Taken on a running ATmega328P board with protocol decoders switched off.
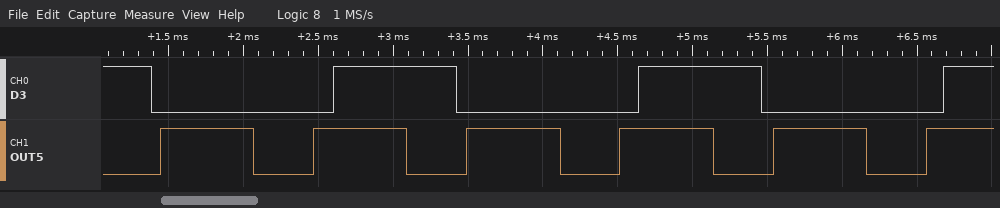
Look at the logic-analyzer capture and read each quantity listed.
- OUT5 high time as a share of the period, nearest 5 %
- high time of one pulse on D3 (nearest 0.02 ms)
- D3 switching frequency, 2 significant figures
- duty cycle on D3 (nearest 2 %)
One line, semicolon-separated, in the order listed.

60 %; 0.82 ms; 490 Hz; 40 %
